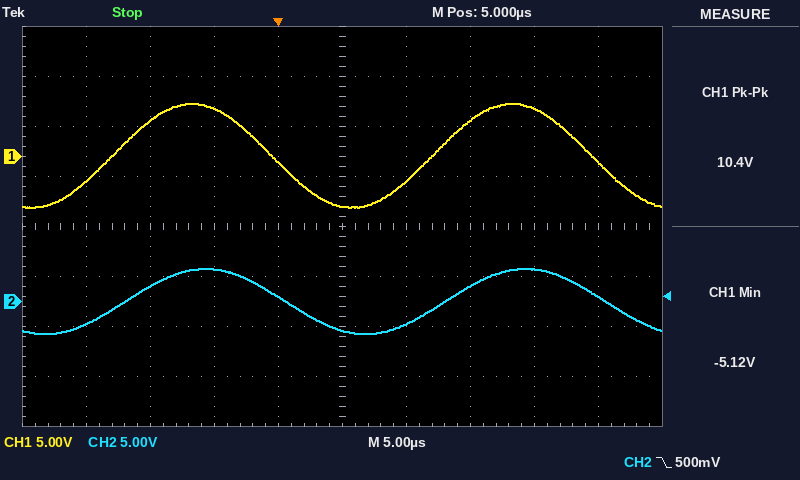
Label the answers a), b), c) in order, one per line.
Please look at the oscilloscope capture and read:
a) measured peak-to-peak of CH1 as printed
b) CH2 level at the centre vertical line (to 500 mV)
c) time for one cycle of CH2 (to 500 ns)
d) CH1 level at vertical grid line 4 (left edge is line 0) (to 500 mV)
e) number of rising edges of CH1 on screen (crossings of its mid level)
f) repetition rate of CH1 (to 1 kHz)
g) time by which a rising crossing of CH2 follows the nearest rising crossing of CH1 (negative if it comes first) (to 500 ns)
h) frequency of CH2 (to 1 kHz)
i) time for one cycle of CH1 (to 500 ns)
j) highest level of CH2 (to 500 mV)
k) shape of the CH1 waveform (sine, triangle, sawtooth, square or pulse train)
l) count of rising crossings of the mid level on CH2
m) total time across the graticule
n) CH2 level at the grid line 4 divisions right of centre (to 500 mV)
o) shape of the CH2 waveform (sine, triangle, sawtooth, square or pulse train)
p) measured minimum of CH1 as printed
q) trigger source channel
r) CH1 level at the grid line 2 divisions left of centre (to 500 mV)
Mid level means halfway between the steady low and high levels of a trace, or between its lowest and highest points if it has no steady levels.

a) 10.4 V
b) -3.0 V
c) 25.0 µs
d) -500 mV
e) 2
f) 40 kHz
g) +1.0 µs
h) 40 kHz
i) 25.0 µs
j) 3.5 V
k) sine
l) 2
m) 50 µs
n) 500 mV
o) sine
p) -5.12 V
q) CH2
r) 5.0 V
